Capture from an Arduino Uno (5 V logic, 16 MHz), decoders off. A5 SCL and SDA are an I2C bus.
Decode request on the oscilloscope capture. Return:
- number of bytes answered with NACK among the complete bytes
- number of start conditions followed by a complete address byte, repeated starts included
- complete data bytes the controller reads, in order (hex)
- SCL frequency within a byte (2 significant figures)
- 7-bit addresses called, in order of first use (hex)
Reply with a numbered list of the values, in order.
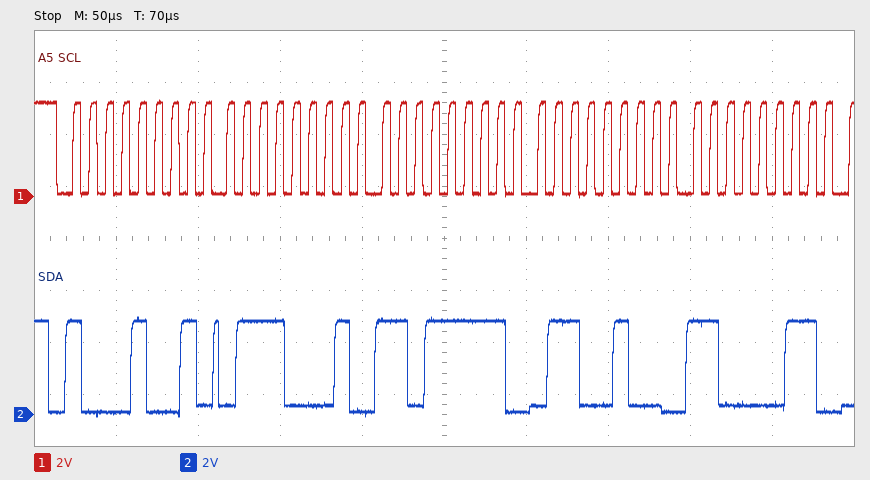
1. 0
2. 1
3. 71 DF 64 C3
4. 100 kHz
5. 0x44
